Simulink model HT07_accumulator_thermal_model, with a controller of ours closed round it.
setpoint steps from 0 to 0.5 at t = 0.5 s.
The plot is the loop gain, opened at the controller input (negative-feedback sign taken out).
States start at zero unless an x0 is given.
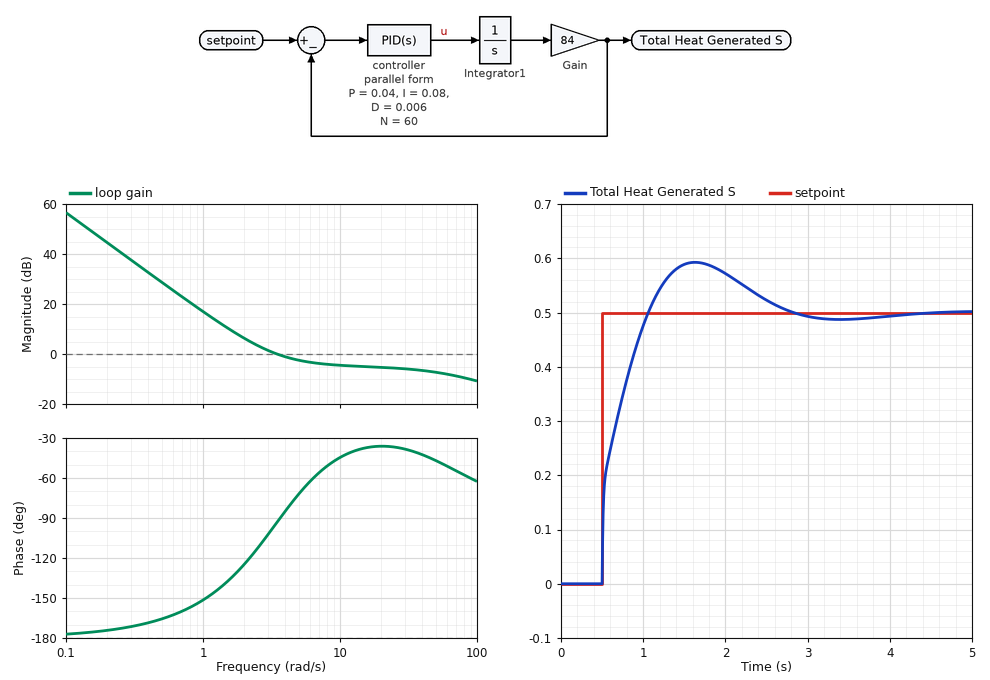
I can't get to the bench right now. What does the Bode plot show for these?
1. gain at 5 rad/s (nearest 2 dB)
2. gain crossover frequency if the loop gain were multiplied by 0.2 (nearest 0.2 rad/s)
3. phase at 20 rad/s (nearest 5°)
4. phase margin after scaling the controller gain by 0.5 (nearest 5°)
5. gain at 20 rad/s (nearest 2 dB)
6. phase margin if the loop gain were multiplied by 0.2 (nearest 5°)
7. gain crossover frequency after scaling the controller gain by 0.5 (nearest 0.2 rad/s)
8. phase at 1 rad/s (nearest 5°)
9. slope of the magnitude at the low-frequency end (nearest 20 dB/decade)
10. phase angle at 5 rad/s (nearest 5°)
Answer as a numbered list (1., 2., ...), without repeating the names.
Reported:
1. -2 dB
2. 1.2 rad/s
3. -35°
4. 55°
5. -6 dB
6. 35°
7. 2.0 rad/s
8. -150°
9. -40 dB/decade
10. -70°
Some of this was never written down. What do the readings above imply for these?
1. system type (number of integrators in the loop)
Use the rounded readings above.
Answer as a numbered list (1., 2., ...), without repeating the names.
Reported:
1. 2
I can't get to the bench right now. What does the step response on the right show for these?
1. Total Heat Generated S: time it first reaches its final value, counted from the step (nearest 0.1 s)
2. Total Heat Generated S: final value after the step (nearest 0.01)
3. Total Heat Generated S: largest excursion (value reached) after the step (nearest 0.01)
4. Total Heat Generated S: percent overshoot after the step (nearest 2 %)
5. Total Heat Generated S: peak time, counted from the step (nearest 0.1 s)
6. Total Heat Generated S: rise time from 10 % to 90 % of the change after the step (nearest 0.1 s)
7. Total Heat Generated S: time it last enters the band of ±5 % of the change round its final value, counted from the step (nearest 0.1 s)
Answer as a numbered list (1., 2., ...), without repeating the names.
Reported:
1. 0.6 s
2. 0.50
3. 0.59
4. 18 %
5. 1.1 s
6. 0.4 s
7. 2.0 s
